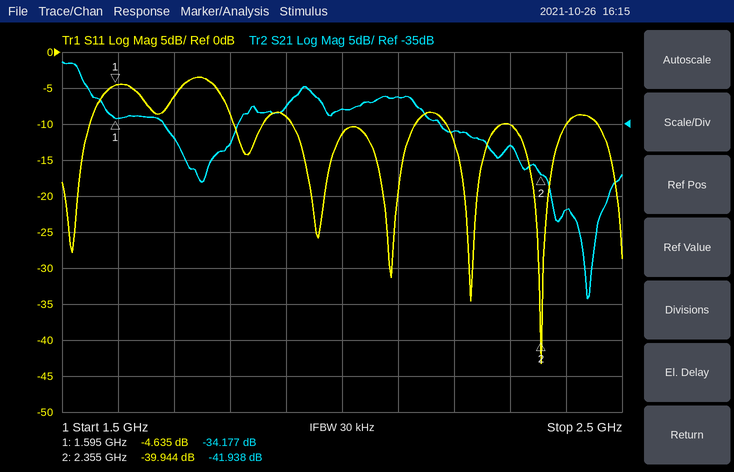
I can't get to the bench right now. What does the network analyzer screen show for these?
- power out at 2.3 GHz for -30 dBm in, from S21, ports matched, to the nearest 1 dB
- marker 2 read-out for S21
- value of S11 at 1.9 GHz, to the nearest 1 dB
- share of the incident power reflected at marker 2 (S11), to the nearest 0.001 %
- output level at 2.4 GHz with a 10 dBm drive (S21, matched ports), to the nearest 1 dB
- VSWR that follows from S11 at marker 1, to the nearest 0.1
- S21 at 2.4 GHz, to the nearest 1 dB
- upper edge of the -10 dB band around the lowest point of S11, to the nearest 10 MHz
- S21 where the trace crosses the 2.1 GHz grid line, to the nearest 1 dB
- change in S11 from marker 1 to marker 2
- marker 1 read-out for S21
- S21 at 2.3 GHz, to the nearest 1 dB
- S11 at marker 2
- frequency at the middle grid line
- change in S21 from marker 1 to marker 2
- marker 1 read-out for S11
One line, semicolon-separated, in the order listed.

-68 dBm; -41.938 dB; -9 dB; 0.010 %; -37 dBm; 3.8; -47 dB; 2.40 GHz; -31 dB; -35.309 dB; -34.177 dB; -38 dB; -39.944 dB; 2 GHz; -7.761 dB; -4.635 dB
